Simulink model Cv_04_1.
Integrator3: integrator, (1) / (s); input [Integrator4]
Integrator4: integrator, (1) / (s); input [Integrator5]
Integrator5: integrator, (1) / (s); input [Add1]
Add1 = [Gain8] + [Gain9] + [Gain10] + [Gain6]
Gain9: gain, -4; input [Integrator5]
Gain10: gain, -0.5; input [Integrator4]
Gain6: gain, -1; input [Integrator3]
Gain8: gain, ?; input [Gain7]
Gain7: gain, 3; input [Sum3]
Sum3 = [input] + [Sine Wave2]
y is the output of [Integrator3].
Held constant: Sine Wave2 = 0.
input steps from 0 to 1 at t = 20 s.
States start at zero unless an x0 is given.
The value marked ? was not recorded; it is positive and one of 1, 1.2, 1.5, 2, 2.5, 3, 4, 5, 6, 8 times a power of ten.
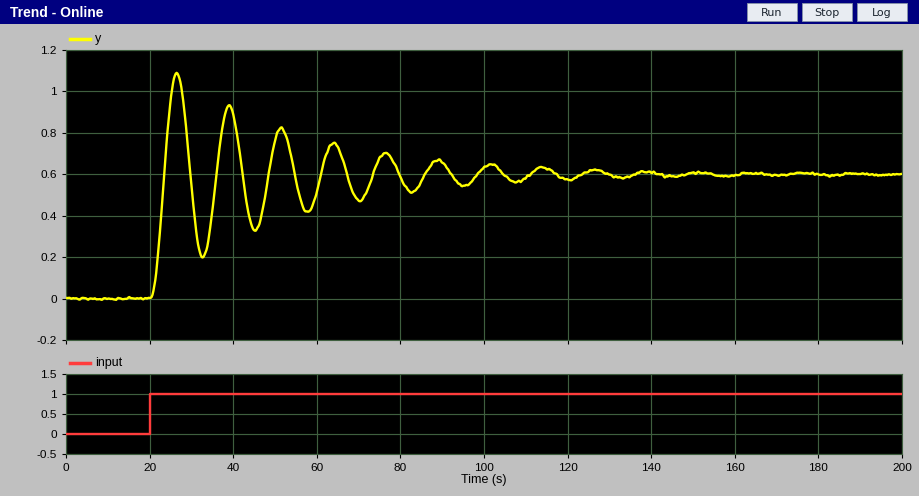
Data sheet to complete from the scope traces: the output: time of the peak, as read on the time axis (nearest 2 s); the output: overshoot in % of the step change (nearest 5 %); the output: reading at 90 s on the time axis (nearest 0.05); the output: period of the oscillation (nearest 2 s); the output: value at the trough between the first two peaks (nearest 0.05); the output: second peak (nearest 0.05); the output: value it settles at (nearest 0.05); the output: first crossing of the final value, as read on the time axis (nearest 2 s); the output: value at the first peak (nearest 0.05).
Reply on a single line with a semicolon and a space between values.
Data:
26 s; 80 %; 0.65; 12 s; 0.20; 0.95; 0.60; 24 s; 1.10
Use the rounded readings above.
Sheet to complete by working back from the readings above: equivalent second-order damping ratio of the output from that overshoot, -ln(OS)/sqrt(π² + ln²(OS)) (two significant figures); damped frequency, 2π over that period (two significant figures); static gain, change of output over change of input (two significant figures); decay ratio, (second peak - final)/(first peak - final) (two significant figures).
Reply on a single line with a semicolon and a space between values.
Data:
0.071; 0.52 rad/s; 0.60; 0.70
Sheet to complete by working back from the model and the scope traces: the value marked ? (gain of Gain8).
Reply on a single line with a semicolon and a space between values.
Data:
0.2
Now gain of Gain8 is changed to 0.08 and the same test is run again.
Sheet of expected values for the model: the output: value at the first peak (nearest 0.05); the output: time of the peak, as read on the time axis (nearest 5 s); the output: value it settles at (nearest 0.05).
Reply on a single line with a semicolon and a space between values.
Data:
0.45; 25 s; 0.25
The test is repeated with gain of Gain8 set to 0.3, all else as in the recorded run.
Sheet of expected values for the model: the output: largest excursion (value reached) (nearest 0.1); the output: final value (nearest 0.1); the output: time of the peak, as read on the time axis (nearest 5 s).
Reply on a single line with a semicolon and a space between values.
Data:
1.6; 0.9; 25 s
